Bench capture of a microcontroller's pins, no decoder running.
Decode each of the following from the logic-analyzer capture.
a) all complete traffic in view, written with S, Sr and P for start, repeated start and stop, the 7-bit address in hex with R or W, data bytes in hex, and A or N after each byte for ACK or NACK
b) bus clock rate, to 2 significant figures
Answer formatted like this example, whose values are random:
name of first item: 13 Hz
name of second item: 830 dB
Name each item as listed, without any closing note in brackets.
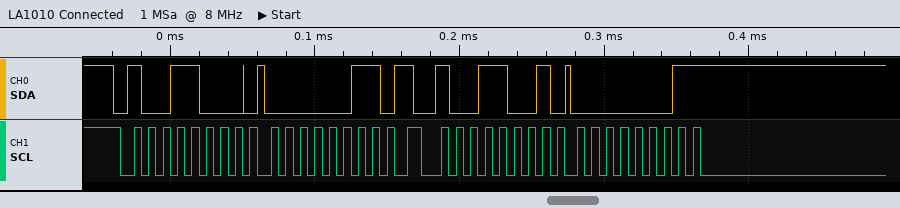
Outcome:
all complete traffic in view, written with S, Sr and P for start, repeated start and stop, the 7-bit address in hex with R or W, data bytes in hex, and A or N after each byte for ACK or NACK: S 4CW A 03 A Sr 4CR A 01 N
bus clock rate, to 2 significant figures: 100 kHz
